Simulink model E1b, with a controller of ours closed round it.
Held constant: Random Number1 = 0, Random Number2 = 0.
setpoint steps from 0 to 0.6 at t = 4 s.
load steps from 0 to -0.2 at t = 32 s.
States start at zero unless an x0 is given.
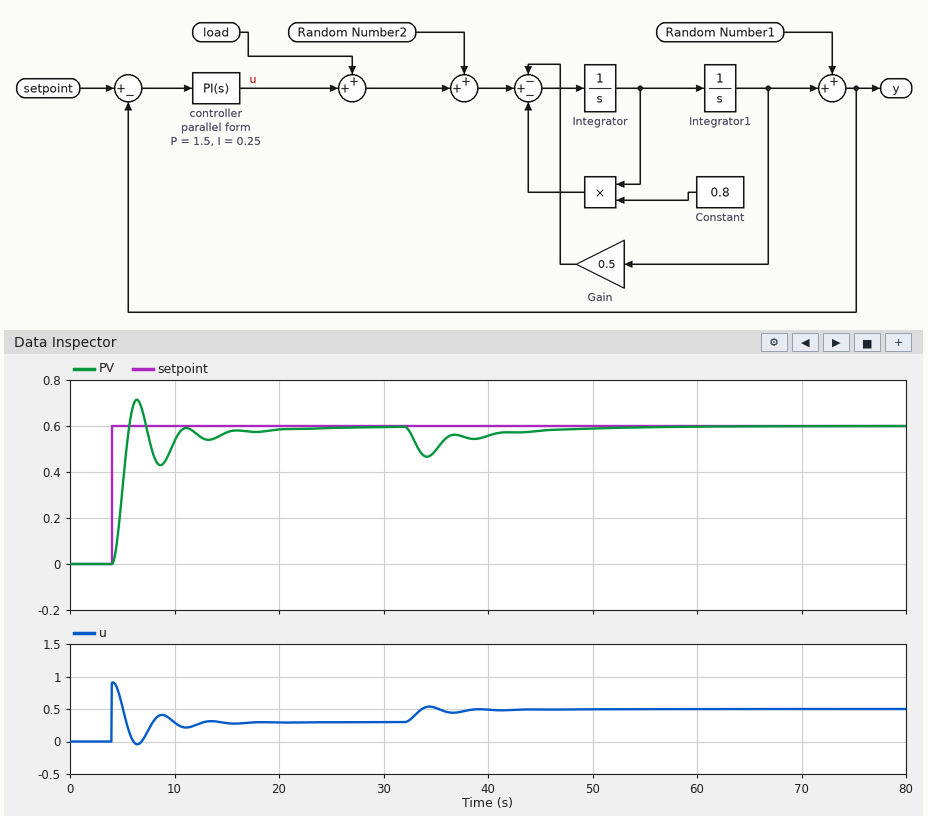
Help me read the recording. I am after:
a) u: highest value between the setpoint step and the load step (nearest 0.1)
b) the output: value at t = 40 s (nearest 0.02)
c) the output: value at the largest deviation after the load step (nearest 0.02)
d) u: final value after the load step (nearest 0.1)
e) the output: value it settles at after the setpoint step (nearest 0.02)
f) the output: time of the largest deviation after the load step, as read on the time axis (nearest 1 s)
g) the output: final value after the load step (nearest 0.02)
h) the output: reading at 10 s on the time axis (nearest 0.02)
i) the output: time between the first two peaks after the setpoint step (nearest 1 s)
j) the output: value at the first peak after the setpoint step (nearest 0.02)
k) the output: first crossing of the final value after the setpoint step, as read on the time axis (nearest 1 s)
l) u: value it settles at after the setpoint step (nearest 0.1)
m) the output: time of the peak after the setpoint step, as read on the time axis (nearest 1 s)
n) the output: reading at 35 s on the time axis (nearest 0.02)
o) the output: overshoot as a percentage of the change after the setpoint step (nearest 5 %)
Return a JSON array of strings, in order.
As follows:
["0.9", "0.56", "0.46", "0.5", "0.60", "34 s", "0.60", "0.54", "5 s", "0.72", "6 s", "0.3", "6 s", "0.50", "20 %"]
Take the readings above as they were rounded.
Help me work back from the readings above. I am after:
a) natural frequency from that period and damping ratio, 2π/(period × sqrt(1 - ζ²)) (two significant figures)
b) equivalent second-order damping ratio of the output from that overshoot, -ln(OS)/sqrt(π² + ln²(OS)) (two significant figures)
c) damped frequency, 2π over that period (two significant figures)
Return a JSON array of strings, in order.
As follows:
["1.4 rad/s", "0.46", "1.3 rad/s"]
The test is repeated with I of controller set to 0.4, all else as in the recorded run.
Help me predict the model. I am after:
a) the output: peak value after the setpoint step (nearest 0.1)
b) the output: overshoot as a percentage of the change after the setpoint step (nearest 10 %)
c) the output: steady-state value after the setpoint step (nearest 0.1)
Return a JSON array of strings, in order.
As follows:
["0.8", "30 %", "0.6"]
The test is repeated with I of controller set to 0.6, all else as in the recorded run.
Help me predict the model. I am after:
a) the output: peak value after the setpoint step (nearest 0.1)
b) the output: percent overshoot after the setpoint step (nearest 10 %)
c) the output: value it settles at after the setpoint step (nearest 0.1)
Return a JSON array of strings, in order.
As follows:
["0.8", "40 %", "0.6"]
